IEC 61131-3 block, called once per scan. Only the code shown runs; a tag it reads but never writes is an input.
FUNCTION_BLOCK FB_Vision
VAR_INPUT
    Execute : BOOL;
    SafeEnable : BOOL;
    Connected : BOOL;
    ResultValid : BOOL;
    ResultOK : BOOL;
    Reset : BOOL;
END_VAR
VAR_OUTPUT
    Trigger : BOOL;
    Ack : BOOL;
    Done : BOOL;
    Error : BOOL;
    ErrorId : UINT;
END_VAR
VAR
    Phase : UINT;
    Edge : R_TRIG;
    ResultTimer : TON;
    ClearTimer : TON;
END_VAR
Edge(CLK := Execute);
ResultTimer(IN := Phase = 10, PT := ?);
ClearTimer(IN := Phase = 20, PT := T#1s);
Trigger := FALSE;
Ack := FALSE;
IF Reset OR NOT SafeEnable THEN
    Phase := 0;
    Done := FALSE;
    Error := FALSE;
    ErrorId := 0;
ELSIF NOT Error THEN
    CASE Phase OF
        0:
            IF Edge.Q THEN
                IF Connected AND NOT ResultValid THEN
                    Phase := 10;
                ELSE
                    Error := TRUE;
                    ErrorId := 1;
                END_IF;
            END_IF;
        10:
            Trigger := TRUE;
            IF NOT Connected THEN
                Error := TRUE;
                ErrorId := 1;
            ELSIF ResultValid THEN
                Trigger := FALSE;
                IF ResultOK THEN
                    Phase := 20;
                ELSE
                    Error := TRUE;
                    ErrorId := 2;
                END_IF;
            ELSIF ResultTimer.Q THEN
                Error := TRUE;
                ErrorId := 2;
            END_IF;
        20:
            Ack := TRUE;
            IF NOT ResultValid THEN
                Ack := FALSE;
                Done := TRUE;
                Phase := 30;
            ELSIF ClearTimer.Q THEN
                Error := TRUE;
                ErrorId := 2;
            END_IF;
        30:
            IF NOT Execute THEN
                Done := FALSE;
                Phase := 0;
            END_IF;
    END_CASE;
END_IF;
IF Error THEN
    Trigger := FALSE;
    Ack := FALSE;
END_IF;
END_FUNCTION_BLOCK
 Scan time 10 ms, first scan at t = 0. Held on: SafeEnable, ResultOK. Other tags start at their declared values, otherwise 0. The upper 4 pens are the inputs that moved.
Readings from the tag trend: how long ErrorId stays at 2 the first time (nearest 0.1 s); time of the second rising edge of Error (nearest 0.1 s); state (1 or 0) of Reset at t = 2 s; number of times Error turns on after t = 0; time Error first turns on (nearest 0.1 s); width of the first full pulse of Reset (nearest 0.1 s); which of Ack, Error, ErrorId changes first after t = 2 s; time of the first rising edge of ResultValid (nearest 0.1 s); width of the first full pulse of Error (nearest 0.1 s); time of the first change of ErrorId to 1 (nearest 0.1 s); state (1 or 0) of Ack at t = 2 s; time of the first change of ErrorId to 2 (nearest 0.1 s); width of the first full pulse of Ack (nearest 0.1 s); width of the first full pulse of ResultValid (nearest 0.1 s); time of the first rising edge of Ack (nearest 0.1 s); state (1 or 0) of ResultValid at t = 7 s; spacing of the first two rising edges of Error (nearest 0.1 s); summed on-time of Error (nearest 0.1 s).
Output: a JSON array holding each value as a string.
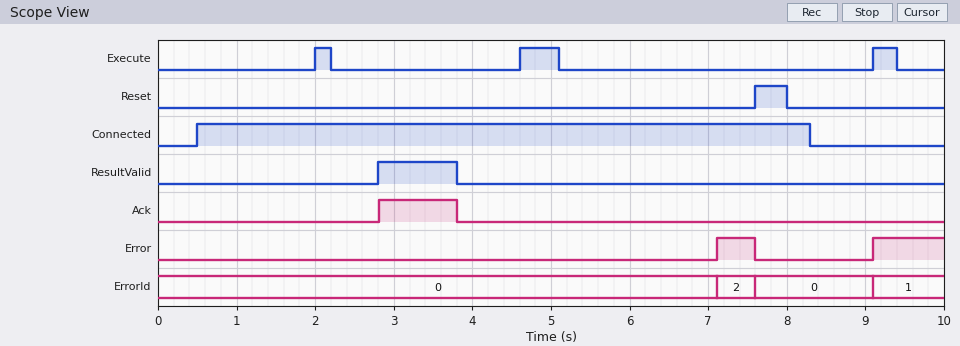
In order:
["0.5 s", "9.1 s", "0", "2", "7.1 s", "0.4 s", "Ack", "2.8 s", "0.5 s", "9.1 s", "0", "7.1 s", "1.0 s", "1.0 s", "2.8 s", "0", "2.0 s", "1.4 s"]
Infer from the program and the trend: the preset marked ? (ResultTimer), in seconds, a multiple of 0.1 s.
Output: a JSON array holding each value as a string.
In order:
["2.5 s"]
